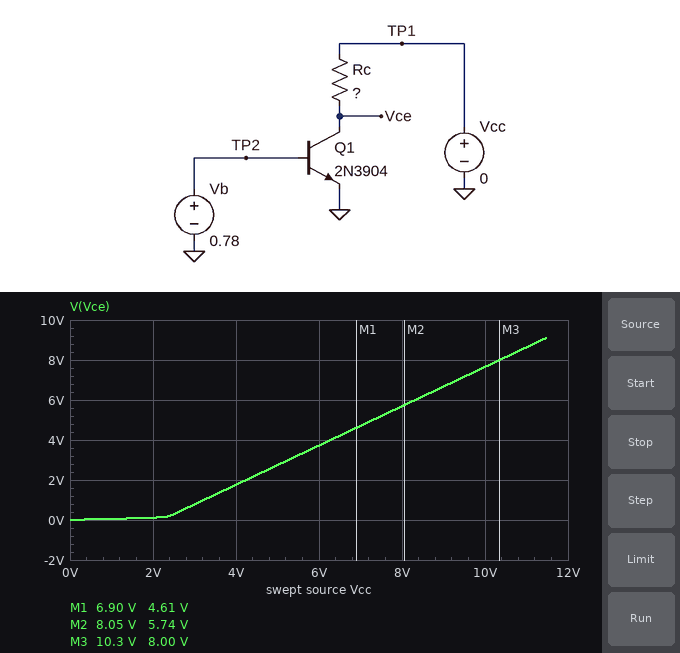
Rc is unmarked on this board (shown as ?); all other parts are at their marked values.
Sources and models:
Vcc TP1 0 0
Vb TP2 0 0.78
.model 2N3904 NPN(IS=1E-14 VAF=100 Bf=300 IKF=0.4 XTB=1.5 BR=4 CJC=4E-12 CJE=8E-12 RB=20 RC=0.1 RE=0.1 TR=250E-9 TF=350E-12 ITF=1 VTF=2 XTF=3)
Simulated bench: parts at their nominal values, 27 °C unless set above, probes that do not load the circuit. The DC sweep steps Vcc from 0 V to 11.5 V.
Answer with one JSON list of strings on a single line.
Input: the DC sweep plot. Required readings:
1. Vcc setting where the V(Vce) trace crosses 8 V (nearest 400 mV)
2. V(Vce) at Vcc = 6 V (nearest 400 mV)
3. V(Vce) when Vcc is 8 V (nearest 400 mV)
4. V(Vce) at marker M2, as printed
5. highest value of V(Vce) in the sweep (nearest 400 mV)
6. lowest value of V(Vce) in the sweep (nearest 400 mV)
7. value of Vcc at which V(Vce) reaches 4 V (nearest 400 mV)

["10.4 V", "3.6 V", "5.6 V", "5.74 V", "9.2 V", "0 V", "6.4 V"]
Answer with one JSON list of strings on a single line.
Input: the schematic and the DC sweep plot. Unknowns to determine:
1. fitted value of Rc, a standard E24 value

["33 Ω"]
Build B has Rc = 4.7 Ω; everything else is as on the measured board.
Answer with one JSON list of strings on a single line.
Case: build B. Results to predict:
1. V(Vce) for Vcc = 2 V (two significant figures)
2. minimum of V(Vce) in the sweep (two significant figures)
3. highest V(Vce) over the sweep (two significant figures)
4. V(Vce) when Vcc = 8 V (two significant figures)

["1.7 V", "4.3 mV", "11 V", "7.7 V"]
